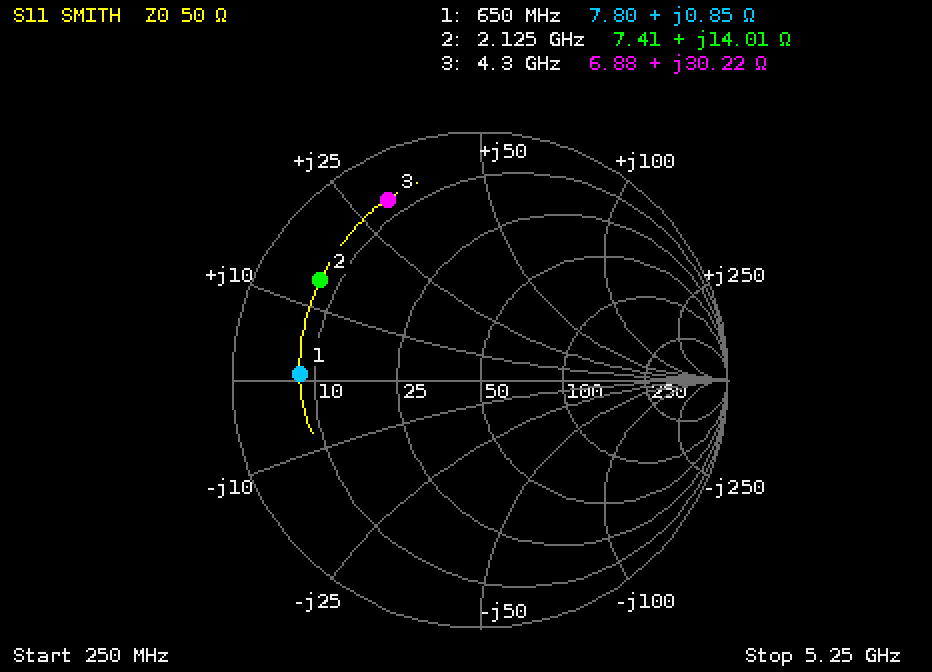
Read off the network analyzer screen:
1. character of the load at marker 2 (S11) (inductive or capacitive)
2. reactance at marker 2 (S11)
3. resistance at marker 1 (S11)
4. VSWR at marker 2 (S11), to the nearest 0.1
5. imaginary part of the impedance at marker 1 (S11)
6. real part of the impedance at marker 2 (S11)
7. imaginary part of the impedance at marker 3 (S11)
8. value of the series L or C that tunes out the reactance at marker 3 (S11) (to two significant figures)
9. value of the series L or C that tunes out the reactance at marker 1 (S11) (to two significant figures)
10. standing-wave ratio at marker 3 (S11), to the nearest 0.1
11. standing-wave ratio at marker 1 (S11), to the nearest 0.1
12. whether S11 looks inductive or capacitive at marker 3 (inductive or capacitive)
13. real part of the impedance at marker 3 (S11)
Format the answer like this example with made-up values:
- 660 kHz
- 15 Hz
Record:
- inductive
- +14.01 Ω
- 7.80 Ω
- 7.3
- +0.85 Ω
- 7.41 Ω
- +30.22 Ω
- 1.2 pF
- 290 pF
- 10.0
- 6.4
- inductive
- 6.88 Ω
